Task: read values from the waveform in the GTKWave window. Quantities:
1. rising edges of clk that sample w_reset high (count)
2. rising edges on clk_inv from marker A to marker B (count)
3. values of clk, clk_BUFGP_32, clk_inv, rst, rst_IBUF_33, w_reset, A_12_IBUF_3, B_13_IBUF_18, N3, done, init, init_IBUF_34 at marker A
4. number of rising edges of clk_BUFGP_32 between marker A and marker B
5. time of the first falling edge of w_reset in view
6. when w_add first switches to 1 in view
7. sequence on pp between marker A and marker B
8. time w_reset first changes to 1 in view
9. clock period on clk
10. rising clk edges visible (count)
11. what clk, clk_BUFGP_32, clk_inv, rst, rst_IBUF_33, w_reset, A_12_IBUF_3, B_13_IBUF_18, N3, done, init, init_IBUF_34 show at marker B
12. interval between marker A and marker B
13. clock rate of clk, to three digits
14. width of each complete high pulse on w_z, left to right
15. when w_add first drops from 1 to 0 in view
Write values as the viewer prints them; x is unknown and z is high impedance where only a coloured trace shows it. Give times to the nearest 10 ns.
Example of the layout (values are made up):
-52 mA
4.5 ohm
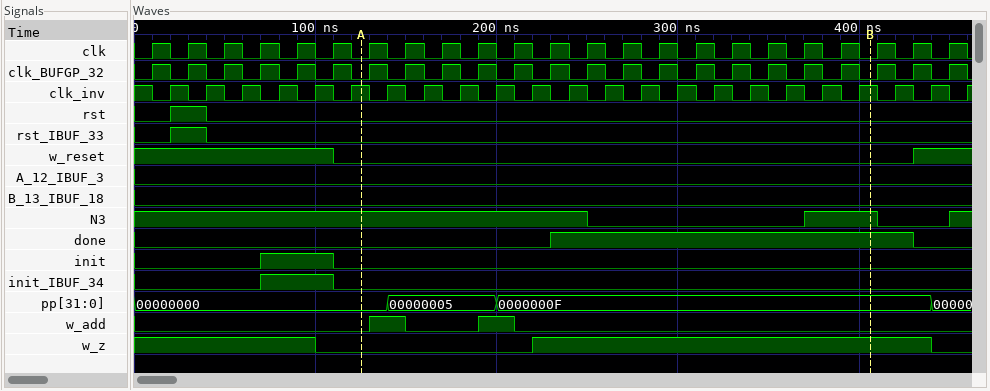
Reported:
7
14
clk=0, clk_BUFGP_32=0, clk_inv=1, rst=0, rst_IBUF_33=0, w_reset=0, A_12_IBUF_3=0, B_13_IBUF_18=0, N3=1, done=0, init=0, init_IBUF_34=0
14
110 ns
130 ns
00000000, 00000005, 0000000F
430 ns
20 ns
23
clk=0, clk_BUFGP_32=0, clk_inv=1, rst=0, rst_IBUF_33=0, w_reset=0, A_12_IBUF_3=0, B_13_IBUF_18=0, N3=1, done=1, init=0, init_IBUF_34=0
280 ns
50.0 MHz
220 ns
150 ns
